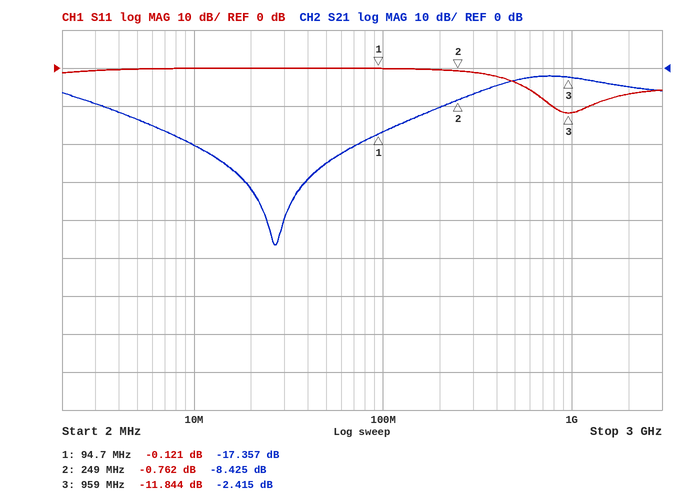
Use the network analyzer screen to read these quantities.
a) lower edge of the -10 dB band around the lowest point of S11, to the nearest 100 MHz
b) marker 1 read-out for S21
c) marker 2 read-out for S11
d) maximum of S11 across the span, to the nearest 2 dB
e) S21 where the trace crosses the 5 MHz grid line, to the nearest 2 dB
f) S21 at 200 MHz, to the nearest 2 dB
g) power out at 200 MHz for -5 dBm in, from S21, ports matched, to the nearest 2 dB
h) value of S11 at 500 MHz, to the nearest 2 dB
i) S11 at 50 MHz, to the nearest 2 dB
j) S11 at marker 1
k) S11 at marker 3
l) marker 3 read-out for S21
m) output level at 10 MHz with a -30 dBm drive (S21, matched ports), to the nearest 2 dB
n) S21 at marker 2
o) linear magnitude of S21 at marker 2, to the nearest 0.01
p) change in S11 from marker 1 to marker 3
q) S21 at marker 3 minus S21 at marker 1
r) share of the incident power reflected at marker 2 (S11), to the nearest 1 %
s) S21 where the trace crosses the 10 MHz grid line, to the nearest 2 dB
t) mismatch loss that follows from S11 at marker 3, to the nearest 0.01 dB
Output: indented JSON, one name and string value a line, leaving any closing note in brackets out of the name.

{
  "lower edge of the -10 dB band around the lowest point of S11, to the nearest 100 MHz": "800 MHz",
  "marker 1 read-out for S21": "-17.357 dB",
  "marker 2 read-out for S11": "-0.762 dB",
  "maximum of S11 across the span, to the nearest 2 dB": "0 dB",
  "S21 where the trace crosses the 5 MHz grid line, to the nearest 2 dB": "-14 dB",
  "S21 at 200 MHz, to the nearest 2 dB": "-10 dB",
  "power out at 200 MHz for -5 dBm in, from S21, ports matched, to the nearest 2 dB": "-16 dBm",
  "value of S11 at 500 MHz, to the nearest 2 dB": "-4 dB",
  "S11 at 50 MHz, to the nearest 2 dB": "0 dB",
  "S11 at marker 1": "-0.121 dB",
  "S11 at marker 3": "-11.844 dB",
  "marker 3 read-out for S21": "-2.415 dB",
  "output level at 10 MHz with a -30 dBm drive (S21, matched ports), to the nearest 2 dB": "-50 dBm",
  "S21 at marker 2": "-8.425 dB",
  "linear magnitude of S21 at marker 2, to the nearest 0.01": "0.38",
  "change in S11 from marker 1 to marker 3": "-11.723 dB",
  "S21 at marker 3 minus S21 at marker 1": "14.942 dB",
  "share of the incident power reflected at marker 2 (S11), to the nearest 1 %": "84 %",
  "S21 where the trace crosses the 10 MHz grid line, to the nearest 2 dB": "-20 dB",
  "mismatch loss that follows from S11 at marker 3, to the nearest 0.01 dB": "0.29 dB"
}
